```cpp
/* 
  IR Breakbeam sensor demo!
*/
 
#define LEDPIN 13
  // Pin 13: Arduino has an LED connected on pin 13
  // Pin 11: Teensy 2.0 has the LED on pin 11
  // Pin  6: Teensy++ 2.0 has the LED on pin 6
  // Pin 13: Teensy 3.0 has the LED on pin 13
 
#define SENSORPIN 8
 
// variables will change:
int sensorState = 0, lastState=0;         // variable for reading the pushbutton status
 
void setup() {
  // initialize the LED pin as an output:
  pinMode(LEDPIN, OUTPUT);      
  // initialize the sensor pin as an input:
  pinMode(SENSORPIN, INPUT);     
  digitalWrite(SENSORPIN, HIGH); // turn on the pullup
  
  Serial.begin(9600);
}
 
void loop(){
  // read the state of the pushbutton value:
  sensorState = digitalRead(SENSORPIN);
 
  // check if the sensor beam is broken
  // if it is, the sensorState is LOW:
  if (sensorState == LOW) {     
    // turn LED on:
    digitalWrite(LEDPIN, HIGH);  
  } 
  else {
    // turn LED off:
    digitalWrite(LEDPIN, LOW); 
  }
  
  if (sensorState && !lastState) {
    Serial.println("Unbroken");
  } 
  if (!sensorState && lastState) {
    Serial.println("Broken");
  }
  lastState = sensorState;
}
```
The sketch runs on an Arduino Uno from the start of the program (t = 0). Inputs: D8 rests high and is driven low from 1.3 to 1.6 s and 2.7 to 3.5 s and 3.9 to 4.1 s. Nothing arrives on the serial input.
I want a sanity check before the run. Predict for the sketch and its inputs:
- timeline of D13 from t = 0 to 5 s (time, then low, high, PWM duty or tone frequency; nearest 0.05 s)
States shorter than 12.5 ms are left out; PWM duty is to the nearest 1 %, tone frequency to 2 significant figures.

0 s low; 1.3 s high; 1.6 s low; 2.7 s high; 3.5 s low; 3.9 s high; 4.1 s low
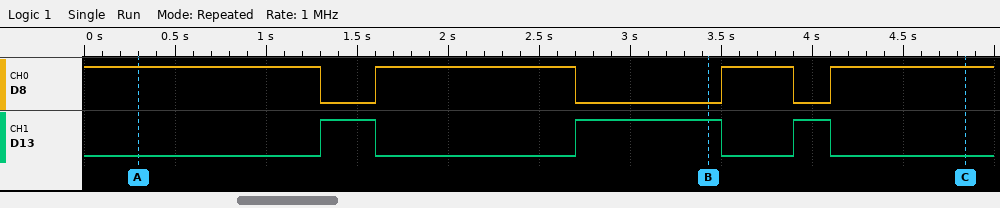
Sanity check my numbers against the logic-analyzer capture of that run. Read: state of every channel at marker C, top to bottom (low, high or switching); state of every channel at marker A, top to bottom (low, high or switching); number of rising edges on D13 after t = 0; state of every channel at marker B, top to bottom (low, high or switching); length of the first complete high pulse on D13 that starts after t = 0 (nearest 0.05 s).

D8 high, D13 low
D8 high, D13 low
3
D8 low, D13 high
0.30 s
